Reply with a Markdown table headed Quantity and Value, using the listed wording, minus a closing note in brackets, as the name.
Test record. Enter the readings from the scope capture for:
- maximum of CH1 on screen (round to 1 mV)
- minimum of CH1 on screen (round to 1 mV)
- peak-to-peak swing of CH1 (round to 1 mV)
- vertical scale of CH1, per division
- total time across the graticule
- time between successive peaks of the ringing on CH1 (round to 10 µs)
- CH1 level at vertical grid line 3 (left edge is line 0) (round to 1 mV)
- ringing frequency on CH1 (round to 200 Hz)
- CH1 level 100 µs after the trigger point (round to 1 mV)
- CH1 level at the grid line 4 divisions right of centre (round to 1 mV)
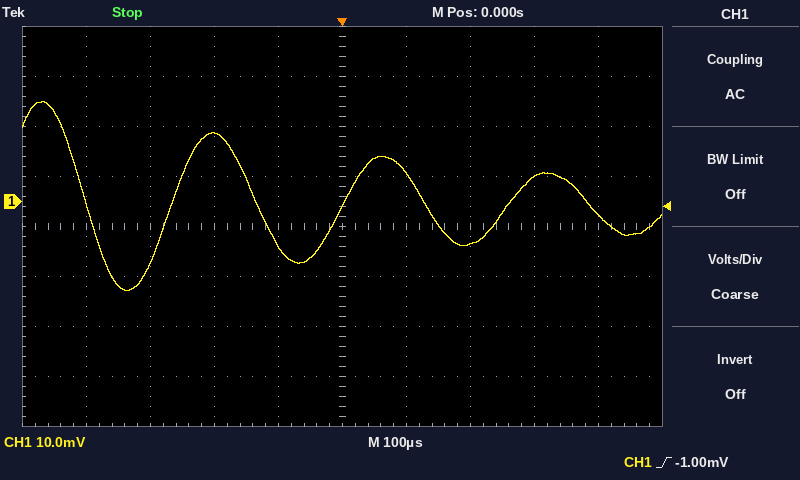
| Quantity | Value |
|---|---|
| maximum of CH1 on screen | 20 mV |
| minimum of CH1 on screen | -18 mV |
| peak-to-peak swing of CH1 | 38 mV |
| vertical scale of CH1, per division | 10 mV |
| total time across the graticule | 1 ms |
| time between successive peaks of the ringing on CH1 | 260 µs |
| CH1 level at vertical grid line 3 (left edge is line 0) | 14 mV |
| ringing frequency on CH1 | 3.8 kHz |
| CH1 level 100 µs after the trigger point | 6 mV |
| CH1 level at the grid line 4 divisions right of centre | -3 mV |
